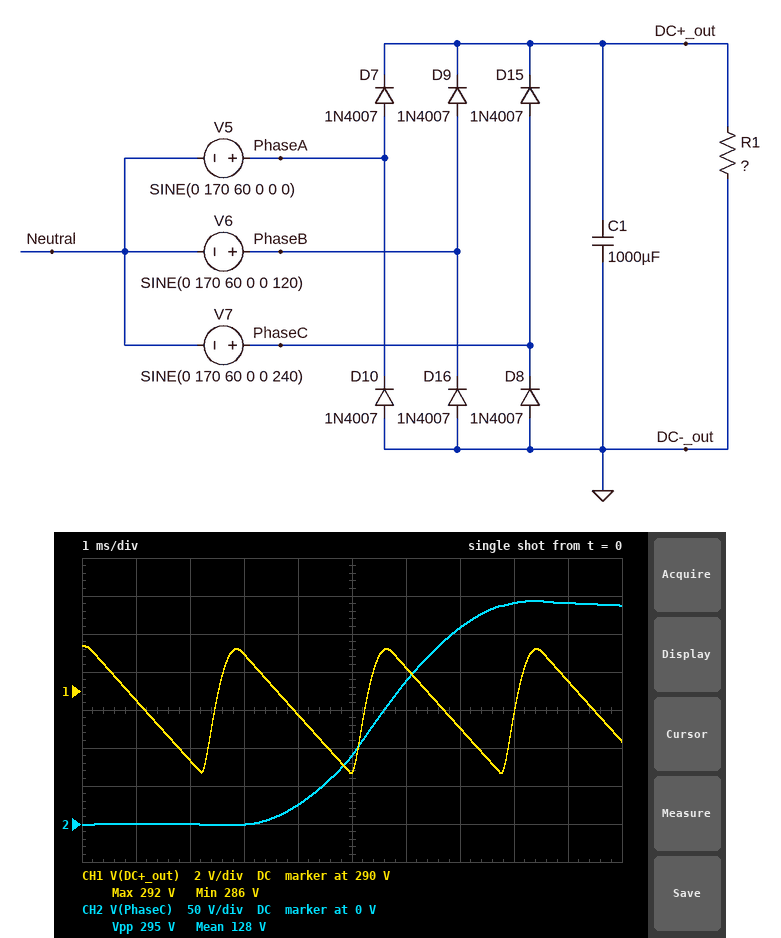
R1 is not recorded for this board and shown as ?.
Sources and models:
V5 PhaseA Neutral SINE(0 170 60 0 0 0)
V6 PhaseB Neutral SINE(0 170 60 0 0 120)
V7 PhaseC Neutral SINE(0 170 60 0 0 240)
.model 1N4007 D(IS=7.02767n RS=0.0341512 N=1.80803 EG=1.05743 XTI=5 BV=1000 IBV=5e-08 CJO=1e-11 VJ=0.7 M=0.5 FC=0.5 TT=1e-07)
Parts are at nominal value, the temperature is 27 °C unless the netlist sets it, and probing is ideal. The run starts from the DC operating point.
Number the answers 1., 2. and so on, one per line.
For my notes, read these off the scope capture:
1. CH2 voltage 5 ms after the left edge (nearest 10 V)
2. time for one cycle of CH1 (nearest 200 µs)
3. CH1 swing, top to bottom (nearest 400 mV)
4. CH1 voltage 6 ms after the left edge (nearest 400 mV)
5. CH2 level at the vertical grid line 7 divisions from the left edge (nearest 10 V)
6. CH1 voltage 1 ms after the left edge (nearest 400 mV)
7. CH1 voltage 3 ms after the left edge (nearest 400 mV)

1. 90 V
2. 2.8 ms
3. 6.8 V
4. 291.2 V
5. 260 V
6. 289.6 V
7. 292.0 V
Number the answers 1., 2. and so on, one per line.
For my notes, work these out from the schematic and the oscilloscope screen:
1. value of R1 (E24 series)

1. 91 Ω
